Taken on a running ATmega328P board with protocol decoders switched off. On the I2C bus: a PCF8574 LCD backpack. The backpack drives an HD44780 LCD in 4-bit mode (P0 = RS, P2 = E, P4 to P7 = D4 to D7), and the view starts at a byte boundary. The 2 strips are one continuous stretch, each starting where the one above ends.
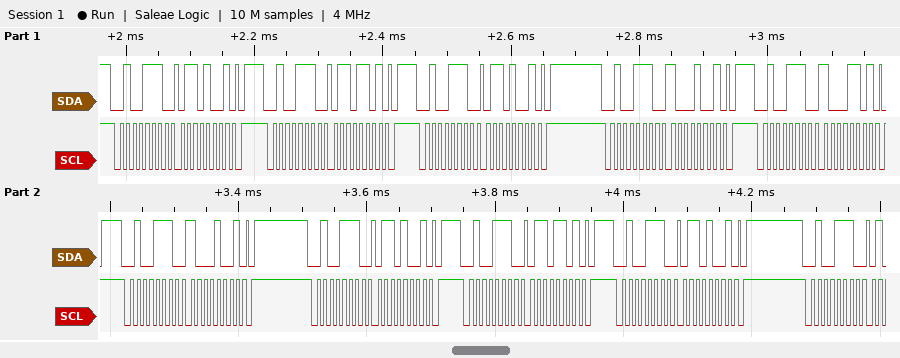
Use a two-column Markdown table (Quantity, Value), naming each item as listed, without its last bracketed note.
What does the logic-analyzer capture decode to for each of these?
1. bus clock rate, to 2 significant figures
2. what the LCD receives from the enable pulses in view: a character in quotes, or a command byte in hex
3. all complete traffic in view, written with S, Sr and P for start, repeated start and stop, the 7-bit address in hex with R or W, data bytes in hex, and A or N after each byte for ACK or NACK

| Quantity | Value |
|---|---|
| bus clock rate, to 2 significant figures | 100 kHz |
| what the LCD receives from the enable pulses in view: a character in quotes, or a command byte in hex | 'h' |
| all complete traffic in view, written with S, Sr and P for start, repeated start and stop, the 7-bit address in hex with R or W, data bytes in hex, and A or N after each byte for ACK or NACK | S 27W A 69 A P S 27W A 6D A P S 27W A 69 A P S 27W A 89 A P S 27W A 8D A P S 27W A 89 A P S 27W A 69 A P S 27W A 6D A P S 27W A 69 A P S 27W A |
